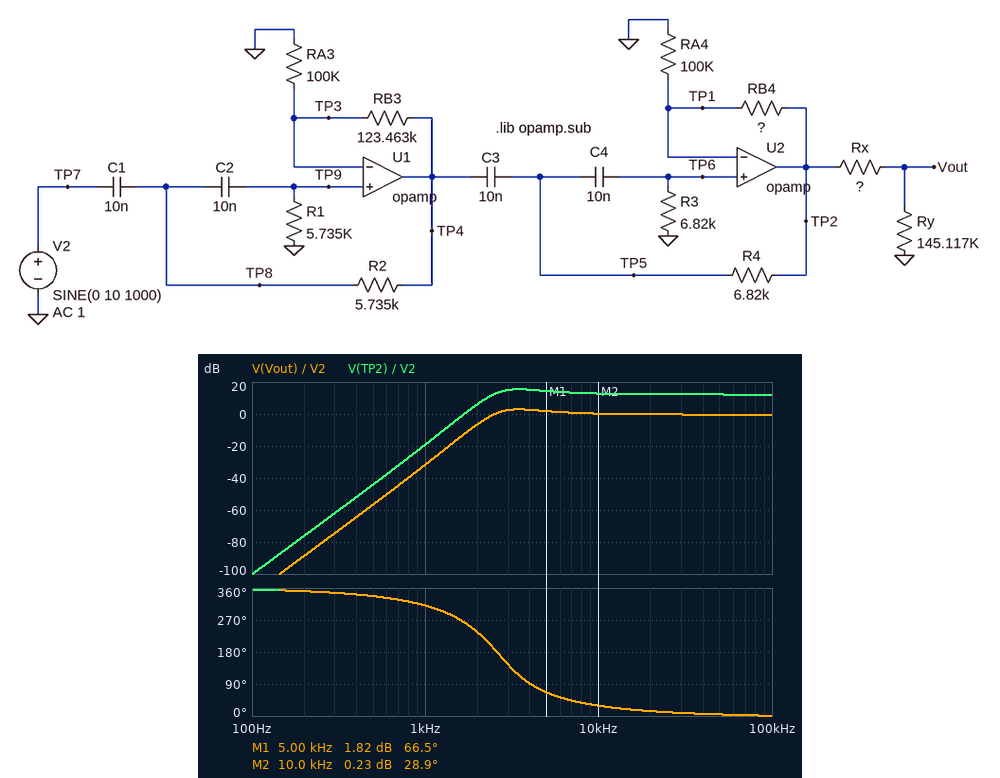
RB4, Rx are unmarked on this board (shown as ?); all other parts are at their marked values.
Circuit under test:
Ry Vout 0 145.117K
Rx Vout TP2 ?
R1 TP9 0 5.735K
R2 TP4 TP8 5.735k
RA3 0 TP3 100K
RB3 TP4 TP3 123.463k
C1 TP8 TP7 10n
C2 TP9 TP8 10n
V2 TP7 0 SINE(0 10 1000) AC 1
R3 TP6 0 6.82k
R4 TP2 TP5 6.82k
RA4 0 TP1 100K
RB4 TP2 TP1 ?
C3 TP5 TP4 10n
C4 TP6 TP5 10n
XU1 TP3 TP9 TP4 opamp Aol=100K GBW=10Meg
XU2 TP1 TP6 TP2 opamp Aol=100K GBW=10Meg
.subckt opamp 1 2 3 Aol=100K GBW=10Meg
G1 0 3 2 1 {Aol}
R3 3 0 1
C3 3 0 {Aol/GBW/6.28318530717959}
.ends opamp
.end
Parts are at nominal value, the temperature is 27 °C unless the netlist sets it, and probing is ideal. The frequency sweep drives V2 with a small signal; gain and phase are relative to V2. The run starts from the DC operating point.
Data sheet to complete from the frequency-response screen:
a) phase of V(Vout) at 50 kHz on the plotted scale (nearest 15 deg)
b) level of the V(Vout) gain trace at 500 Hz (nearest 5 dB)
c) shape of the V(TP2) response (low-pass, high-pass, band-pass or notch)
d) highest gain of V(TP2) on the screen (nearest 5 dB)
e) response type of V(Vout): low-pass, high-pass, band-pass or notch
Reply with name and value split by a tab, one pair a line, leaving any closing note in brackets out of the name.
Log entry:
phase of V(Vout) at 50 kHz on the plotted scale	0 deg
level of the V(Vout) gain trace at 500 Hz	-55 dB
shape of the V(TP2) response	high-pass
highest gain of V(TP2) on the screen	15 dB
response type of V(Vout): low-pass, high-pass, band-pass or notch	high-pass
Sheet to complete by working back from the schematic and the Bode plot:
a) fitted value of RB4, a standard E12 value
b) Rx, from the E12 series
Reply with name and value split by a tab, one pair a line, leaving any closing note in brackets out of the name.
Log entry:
fitted value of RB4, a standard E12 value	82 kΩ
Rx, from the E12 series	470 kΩ
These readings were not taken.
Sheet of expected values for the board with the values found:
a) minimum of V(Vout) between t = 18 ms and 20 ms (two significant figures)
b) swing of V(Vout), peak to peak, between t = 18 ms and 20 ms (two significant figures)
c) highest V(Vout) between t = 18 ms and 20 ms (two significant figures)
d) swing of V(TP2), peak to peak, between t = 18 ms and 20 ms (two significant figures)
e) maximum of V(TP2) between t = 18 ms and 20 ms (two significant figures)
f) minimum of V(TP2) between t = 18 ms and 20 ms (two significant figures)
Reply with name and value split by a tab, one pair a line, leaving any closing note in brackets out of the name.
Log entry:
minimum of V(Vout) between t = 18 ms and 20 ms	-260 mV
swing of V(Vout), peak to peak, between t = 18 ms and 20 ms	520 mV
highest V(Vout) between t = 18 ms and 20 ms	260 mV
swing of V(TP2), peak to peak, between t = 18 ms and 20 ms	2.2 V
maximum of V(TP2) between t = 18 ms and 20 ms	1.1 V
minimum of V(TP2) between t = 18 ms and 20 ms	-1.1 V
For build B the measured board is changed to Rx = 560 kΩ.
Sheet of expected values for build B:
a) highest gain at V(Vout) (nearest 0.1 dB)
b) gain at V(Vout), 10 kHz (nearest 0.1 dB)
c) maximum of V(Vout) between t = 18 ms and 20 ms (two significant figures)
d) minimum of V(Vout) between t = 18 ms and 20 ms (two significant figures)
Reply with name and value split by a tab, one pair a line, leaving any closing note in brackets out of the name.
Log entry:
highest gain at V(Vout)	1.7 dB
gain at V(Vout), 10 kHz	-1.0 dB
maximum of V(Vout) between t = 18 ms and 20 ms	230 mV
minimum of V(Vout) between t = 18 ms and 20 ms	-230 mV
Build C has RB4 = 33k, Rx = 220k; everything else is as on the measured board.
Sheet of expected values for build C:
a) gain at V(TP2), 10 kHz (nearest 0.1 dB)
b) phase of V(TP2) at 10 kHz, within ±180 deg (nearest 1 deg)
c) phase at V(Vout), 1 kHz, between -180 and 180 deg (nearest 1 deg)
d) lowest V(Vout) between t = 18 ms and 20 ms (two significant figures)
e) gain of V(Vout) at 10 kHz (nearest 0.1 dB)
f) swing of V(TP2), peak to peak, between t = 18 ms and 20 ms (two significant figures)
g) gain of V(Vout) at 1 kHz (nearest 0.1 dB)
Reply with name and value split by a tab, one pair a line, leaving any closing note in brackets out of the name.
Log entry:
gain at V(TP2), 10 kHz	9.7 dB
phase of V(TP2) at 10 kHz, within ±180 deg	35 deg
phase at V(Vout), 1 kHz, between -180 and 180 deg	-59 deg
lowest V(Vout) between t = 18 ms and 20 ms	-280 mV
gain of V(Vout) at 10 kHz	1.7 dB
swing of V(TP2), peak to peak, between t = 18 ms and 20 ms	1.4 V
gain of V(Vout) at 1 kHz	-30.9 dB
